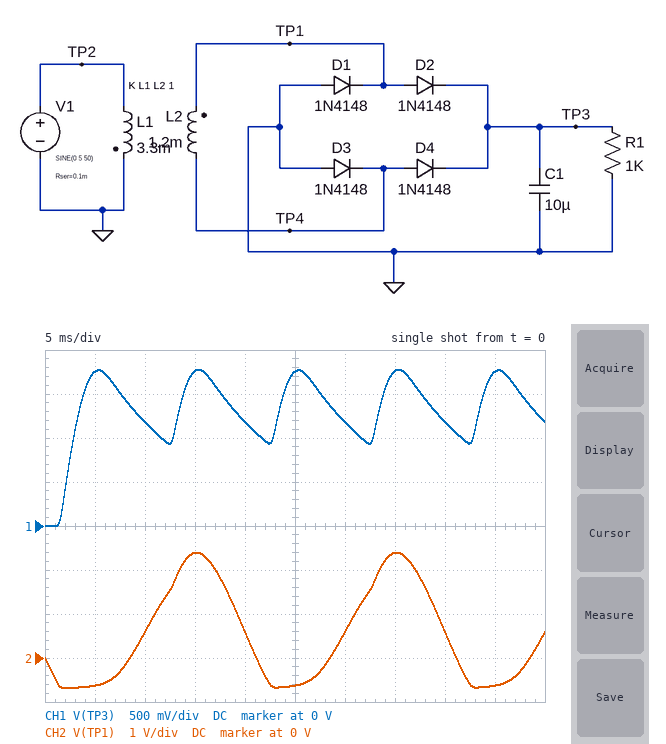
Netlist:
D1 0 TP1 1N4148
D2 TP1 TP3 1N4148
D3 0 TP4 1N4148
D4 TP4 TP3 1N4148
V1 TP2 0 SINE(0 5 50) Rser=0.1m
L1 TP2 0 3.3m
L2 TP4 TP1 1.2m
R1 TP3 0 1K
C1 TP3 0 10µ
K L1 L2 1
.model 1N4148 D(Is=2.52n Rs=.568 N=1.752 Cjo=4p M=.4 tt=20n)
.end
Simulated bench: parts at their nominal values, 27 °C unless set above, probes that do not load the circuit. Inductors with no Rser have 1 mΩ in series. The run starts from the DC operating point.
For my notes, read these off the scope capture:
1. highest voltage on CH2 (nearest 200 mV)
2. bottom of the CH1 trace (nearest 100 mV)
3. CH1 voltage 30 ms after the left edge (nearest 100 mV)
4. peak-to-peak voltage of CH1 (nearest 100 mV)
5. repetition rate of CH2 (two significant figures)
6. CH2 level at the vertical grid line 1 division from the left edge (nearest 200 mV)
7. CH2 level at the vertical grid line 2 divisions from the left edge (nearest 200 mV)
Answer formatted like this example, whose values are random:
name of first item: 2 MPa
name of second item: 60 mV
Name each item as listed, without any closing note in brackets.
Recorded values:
highest voltage on CH2: 2.4 V
bottom of the CH1 trace: 0 V
CH1 voltage 30 ms after the left edge: 1.2 V
peak-to-peak voltage of CH1: 1.8 V
repetition rate of CH2: 50 Hz
CH2 level at the vertical grid line 1 division from the left edge: -600 mV
CH2 level at the vertical grid line 2 divisions from the left edge: 600 mV
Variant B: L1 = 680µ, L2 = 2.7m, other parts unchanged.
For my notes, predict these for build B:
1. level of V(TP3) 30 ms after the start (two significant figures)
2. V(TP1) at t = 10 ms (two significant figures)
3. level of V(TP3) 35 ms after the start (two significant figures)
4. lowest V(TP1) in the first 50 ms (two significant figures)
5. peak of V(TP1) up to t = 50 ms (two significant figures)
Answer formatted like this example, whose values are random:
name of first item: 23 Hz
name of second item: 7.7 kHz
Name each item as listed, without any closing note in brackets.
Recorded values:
level of V(TP3) 30 ms after the start: 5.5 V
V(TP1) at t = 10 ms: 2.8 V
level of V(TP3) 35 ms after the start: 8.6 V
lowest V(TP1) in the first 50 ms: -760 mV
peak of V(TP1) up to t = 50 ms: 9.3 V
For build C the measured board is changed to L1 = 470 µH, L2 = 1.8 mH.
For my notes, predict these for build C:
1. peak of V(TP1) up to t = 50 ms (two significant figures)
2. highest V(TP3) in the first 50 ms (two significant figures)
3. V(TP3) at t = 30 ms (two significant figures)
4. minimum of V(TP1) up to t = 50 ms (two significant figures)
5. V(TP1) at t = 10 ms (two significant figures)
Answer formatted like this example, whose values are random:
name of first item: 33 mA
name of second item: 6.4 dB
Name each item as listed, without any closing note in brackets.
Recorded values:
peak of V(TP1) up to t = 50 ms: 9.2 V
highest V(TP3) in the first 50 ms: 8.5 V
V(TP3) at t = 30 ms: 5.4 V
minimum of V(TP1) up to t = 50 ms: -760 mV
V(TP1) at t = 10 ms: 2.8 V
